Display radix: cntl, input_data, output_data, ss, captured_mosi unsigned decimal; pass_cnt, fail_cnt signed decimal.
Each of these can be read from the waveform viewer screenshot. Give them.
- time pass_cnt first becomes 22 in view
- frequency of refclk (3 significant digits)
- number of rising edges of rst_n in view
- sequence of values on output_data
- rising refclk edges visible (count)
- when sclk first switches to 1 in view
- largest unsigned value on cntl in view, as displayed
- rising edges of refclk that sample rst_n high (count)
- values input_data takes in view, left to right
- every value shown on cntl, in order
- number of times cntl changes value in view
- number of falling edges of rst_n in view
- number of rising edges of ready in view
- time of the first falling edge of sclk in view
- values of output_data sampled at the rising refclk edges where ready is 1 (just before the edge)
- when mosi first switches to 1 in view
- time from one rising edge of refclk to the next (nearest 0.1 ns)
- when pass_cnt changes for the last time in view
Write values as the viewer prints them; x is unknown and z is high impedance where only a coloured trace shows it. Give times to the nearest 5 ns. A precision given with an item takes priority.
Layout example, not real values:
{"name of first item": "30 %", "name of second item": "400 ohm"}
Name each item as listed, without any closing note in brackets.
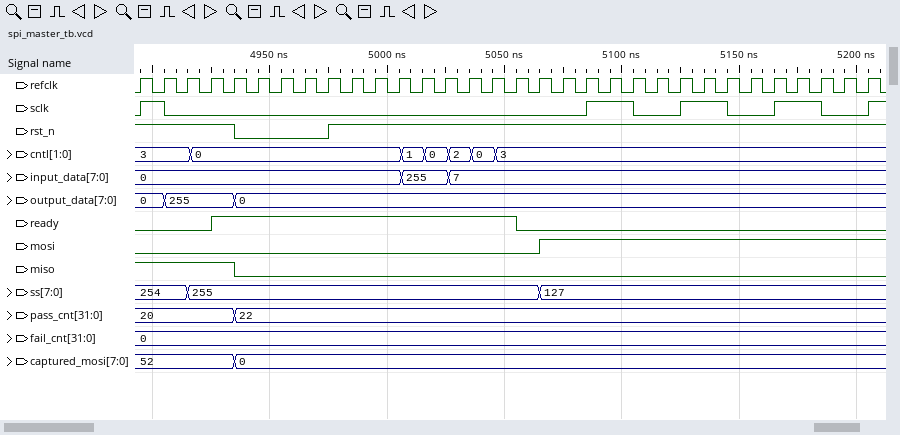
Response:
{"time pass_cnt first becomes 22 in view": "4935 ns", "frequency of refclk": "100 MHz", "number of rising edges of rst_n in view": "1", "sequence of values on output_data": "0, 255, 0", "rising refclk edges visible": "32", "when sclk first switches to 1 in view": "4895 ns", "largest unsigned value on cntl in view, as displayed": "3", "rising edges of refclk that sample rst_n high": "28", "values input_data takes in view, left to right": "0, 255, 7", "every value shown on cntl, in order": "3, 0, 1, 0, 2, 0, 3", "number of times cntl changes value in view": "6", "number of falling edges of rst_n in view": "1", "number of rising edges of ready in view": "1", "time of the first falling edge of sclk in view": "4905 ns", "values of output_data sampled at the rising refclk edges where ready is 1": "255, 0, 0, 0, 0, 0, 0, 0, 0, 0, 0, 0, 0", "when mosi first switches to 1 in view": "5065 ns", "time from one rising edge of refclk to the next": "10 ns", "when pass_cnt changes for the last time in view": "4935 ns"}
